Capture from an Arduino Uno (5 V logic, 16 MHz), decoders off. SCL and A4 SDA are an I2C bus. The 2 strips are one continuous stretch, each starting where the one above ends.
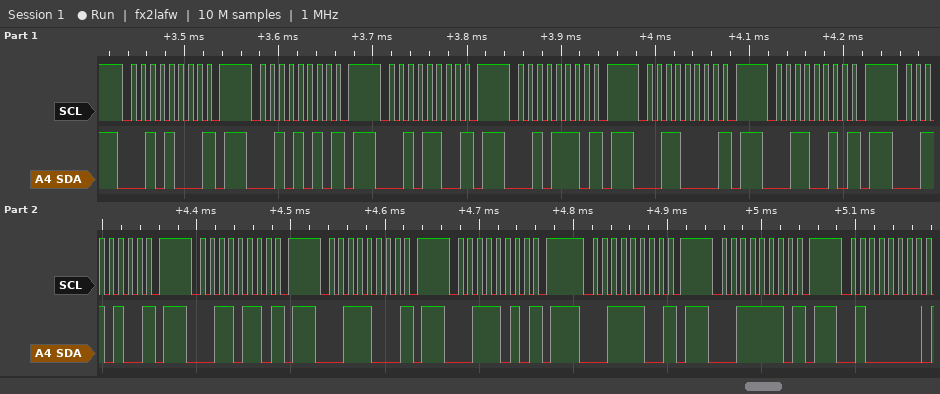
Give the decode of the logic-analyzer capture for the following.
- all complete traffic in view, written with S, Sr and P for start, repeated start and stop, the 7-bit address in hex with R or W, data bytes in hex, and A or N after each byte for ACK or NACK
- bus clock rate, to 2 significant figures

S 14W N P S 15W N P S 16W N P S 17W N P S 18W N P S 19W N P S 1AW N P S 1BW N P S 1CW N P S 1DW N P S 1EW N P S 1FW N P S 20W A
100 kHz
